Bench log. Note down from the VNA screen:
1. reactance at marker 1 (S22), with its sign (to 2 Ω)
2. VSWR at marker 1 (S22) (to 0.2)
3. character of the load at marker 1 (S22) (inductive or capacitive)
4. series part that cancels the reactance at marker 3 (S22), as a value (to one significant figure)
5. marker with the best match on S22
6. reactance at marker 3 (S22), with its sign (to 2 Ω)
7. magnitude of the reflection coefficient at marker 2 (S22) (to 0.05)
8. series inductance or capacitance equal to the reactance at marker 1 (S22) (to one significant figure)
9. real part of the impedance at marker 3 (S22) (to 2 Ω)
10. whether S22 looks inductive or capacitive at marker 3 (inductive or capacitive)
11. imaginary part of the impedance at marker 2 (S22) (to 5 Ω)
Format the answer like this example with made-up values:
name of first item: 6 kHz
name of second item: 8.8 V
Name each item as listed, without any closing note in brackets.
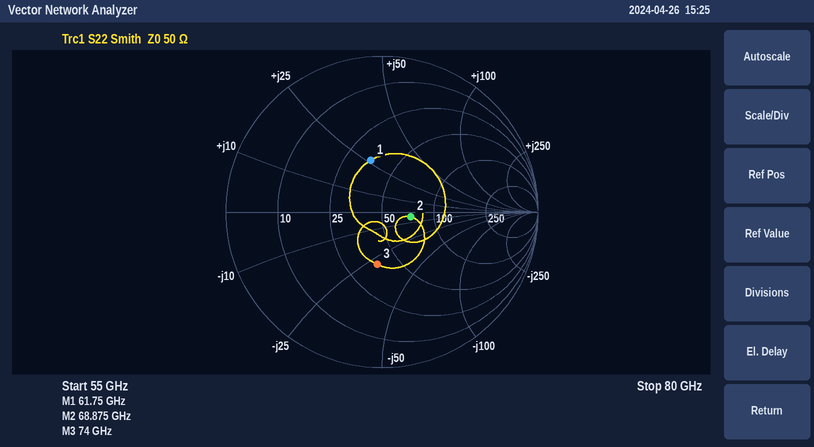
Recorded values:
reactance at marker 1 (S22), with its sign: +26 Ω
VSWR at marker 1 (S22): 2.0
character of the load at marker 1 (S22): inductive
series part that cancels the reactance at marker 3 (S22), as a value: 60 pH
marker with the best match on S22: marker 2
reactance at marker 3 (S22), with its sign: -28 Ω
magnitude of the reflection coefficient at marker 2 (S22): 0.20
series inductance or capacitance equal to the reactance at marker 1 (S22): 70 pH
real part of the impedance at marker 3 (S22): 38 Ω
whether S22 looks inductive or capacitive at marker 3: capacitive
imaginary part of the impedance at marker 2 (S22): -5 Ω
